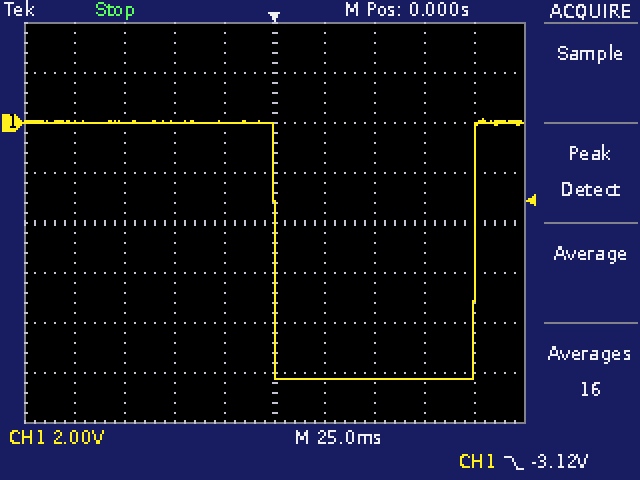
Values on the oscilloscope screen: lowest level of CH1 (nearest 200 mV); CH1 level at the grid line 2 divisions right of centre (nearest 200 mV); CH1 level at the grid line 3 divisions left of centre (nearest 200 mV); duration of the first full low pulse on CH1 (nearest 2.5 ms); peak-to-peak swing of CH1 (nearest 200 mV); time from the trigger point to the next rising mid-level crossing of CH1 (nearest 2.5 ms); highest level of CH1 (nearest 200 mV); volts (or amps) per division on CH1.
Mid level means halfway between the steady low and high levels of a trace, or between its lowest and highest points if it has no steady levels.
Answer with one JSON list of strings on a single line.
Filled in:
["-10.2 V", "-10.2 V", "0.0 V", "100.0 ms", "10.4 V", "100.0 ms", "200 mV", "2 V"]
